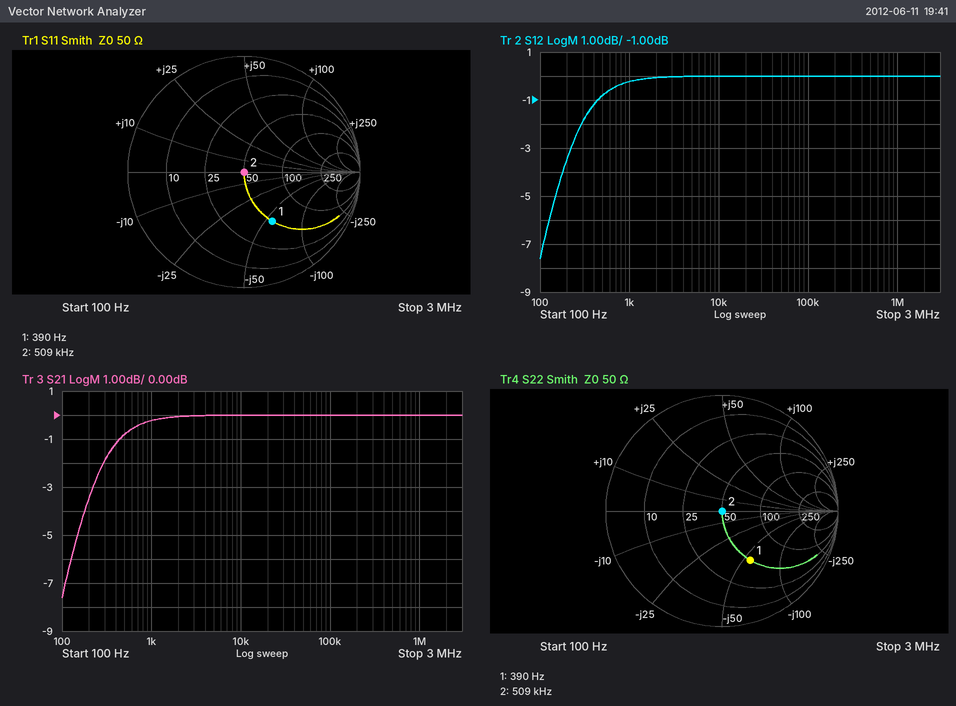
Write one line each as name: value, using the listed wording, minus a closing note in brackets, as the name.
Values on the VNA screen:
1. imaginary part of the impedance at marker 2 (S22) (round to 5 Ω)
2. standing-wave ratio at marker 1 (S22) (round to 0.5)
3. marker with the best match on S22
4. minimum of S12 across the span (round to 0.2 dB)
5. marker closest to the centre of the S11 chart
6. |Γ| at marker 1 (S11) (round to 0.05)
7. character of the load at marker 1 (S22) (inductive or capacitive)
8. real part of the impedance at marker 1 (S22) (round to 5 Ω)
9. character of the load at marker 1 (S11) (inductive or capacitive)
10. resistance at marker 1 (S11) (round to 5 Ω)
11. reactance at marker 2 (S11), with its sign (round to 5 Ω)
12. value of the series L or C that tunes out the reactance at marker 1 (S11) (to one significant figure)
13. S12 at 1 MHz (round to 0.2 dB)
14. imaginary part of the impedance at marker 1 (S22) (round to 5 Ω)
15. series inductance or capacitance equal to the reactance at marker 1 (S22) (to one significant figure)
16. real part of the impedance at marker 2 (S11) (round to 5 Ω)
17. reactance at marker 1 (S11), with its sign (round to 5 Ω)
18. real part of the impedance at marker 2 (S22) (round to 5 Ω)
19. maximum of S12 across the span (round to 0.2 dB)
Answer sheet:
imaginary part of the impedance at marker 2 (S22): 0 Ω
standing-wave ratio at marker 1 (S22): 3.0
marker with the best match on S22: marker 2
minimum of S12 across the span: -7.6 dB
marker closest to the centre of the S11 chart: marker 2
|Γ| at marker 1 (S11): 0.50
character of the load at marker 1 (S22): capacitive
real part of the impedance at marker 1 (S22): 50 Ω
character of the load at marker 1 (S11): capacitive
resistance at marker 1 (S11): 50 Ω
reactance at marker 2 (S11), with its sign: 0 Ω
value of the series L or C that tunes out the reactance at marker 1 (S11): 20 mH
S12 at 1 MHz: 0.0 dB
imaginary part of the impedance at marker 1 (S22): -55 Ω
series inductance or capacitance equal to the reactance at marker 1 (S22): 7 µF
real part of the impedance at marker 2 (S11): 50 Ω
reactance at marker 1 (S11), with its sign: -55 Ω
real part of the impedance at marker 2 (S22): 50 Ω
maximum of S12 across the span: 0.0 dB
